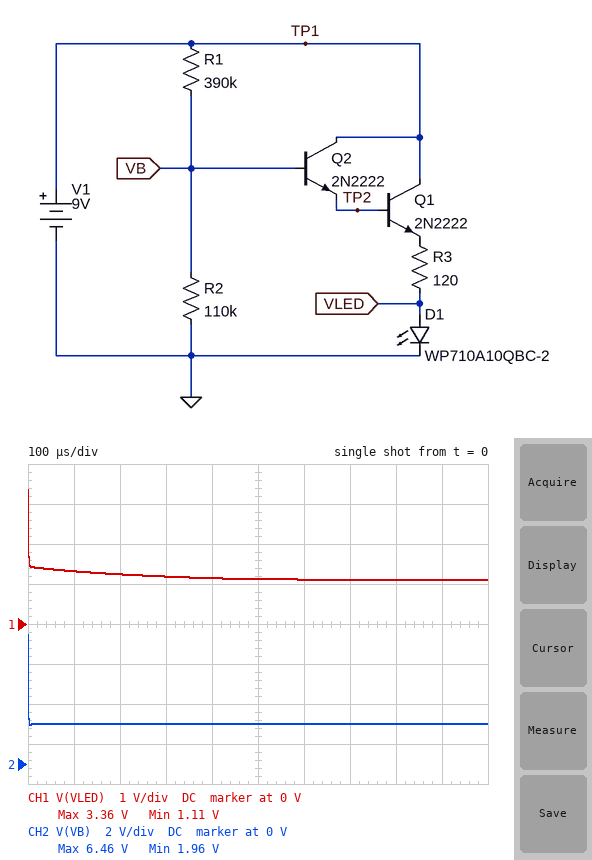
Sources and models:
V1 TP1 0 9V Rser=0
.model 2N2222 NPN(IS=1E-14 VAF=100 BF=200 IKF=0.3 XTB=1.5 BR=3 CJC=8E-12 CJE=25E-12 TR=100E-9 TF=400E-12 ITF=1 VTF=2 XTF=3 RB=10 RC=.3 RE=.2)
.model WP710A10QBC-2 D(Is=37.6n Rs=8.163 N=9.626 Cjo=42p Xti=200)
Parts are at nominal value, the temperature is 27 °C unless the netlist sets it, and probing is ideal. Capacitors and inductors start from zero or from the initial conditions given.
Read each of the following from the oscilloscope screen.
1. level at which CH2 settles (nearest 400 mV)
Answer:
2.0 V
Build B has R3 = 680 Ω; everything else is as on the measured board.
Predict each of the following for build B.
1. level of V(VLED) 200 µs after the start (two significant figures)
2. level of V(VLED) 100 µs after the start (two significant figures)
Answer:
1.3 V
1.4 V
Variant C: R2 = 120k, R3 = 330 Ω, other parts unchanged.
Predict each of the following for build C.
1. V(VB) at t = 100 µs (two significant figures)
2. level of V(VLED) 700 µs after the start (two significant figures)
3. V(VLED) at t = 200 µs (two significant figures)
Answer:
2.1 V
1.2 V
1.3 V
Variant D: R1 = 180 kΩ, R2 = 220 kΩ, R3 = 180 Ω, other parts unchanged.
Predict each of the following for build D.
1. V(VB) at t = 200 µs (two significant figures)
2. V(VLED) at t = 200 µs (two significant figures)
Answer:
4.9 V
2.9 V
